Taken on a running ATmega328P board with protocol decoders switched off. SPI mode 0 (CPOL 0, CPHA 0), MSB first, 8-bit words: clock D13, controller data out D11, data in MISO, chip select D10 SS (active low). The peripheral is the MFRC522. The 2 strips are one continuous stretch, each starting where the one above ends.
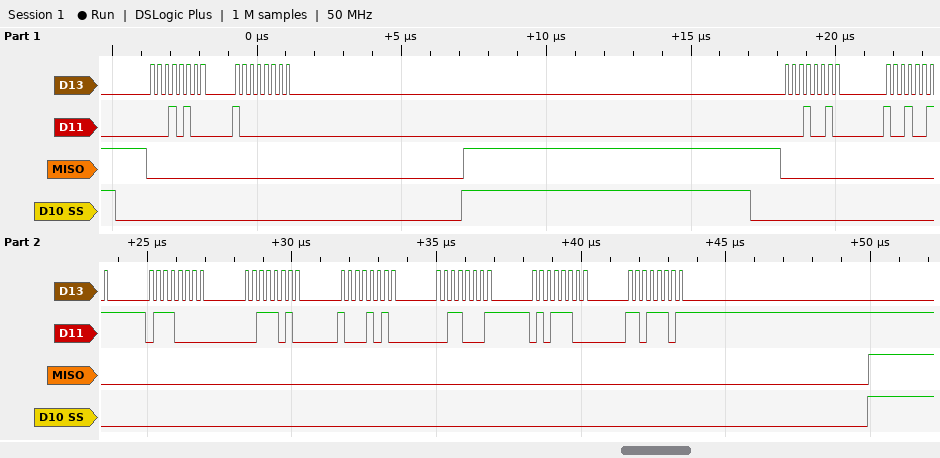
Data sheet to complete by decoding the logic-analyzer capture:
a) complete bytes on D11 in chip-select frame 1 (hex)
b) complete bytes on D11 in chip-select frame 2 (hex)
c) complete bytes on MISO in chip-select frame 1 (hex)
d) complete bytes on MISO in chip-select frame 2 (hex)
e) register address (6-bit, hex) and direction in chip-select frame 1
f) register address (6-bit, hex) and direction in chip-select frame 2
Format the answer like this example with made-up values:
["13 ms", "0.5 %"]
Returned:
["14 80", "12 93 70 3A 8A 31 5C DD", "00 00", "00 00 00 00 00 00 00 00", "0x0A write", "0x09 write"]
